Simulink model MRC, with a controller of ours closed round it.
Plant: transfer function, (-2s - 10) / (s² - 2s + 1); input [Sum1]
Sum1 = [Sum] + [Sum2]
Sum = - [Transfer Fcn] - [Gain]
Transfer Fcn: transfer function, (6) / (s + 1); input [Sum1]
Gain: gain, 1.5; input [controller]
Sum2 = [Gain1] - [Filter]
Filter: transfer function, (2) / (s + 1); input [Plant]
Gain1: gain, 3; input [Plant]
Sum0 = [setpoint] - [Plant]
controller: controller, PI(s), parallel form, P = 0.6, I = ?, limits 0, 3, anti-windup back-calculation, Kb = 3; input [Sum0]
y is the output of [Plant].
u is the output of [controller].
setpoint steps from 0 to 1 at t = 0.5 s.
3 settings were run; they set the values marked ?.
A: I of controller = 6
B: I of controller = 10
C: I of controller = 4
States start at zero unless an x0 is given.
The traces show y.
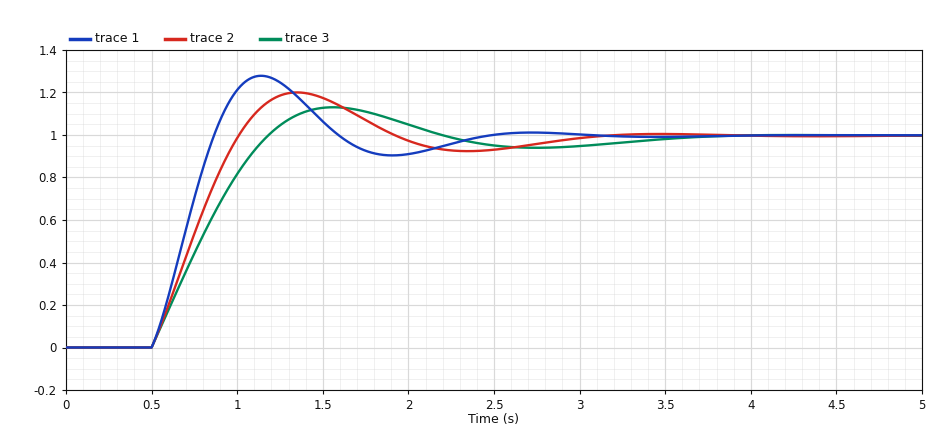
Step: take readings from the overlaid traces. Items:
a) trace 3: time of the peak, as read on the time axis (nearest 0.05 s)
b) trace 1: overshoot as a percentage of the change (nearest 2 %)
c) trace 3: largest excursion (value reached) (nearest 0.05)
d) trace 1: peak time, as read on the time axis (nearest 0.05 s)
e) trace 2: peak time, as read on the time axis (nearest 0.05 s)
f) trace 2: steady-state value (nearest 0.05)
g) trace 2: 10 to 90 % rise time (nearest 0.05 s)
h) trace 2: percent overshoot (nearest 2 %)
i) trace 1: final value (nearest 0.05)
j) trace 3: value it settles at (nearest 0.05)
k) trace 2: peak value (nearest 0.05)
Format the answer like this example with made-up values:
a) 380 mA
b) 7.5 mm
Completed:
a) 1.55 s
b) 28 %
c) 1.15
d) 1.15 s
e) 1.35 s
f) 1.00
g) 0.40 s
h) 20 %
i) 1.00
j) 1.00
k) 1.20
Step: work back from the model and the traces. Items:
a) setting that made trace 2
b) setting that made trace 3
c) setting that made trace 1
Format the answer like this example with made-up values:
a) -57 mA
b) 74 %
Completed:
a) A
b) C
c) B
